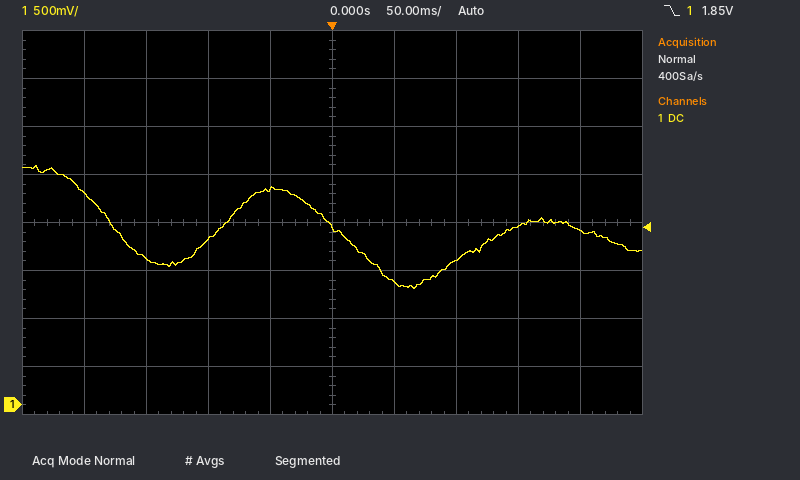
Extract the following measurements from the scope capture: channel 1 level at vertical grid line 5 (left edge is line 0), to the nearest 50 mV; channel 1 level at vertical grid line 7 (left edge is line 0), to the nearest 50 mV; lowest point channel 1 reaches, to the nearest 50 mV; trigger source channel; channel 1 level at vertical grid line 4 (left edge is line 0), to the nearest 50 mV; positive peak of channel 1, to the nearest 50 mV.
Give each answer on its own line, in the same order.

1.85 V
1.50 V
1.20 V
channel 1
2.25 V
2.50 V
